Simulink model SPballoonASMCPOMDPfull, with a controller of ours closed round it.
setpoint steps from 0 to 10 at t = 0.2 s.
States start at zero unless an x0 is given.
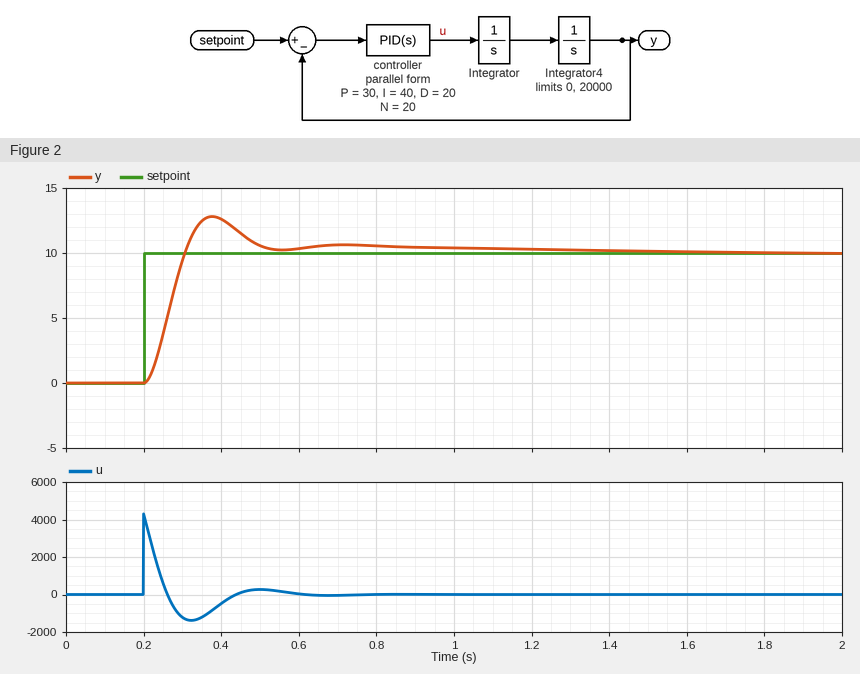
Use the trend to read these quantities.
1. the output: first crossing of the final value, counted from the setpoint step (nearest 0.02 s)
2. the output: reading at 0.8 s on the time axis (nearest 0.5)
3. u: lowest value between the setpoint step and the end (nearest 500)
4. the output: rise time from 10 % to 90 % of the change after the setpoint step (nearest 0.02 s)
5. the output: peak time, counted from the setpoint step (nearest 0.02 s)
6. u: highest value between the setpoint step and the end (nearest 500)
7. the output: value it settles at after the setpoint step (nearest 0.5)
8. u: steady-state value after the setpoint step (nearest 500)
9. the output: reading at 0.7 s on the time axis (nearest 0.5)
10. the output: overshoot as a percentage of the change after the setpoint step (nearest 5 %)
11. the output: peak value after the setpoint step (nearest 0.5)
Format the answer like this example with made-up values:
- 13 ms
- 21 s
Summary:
- 0.10 s
- 10.5
- -1500
- 0.08 s
- 0.18 s
- 4500
- 10.0
- 0
- 10.5
- 30 %
- 13.0
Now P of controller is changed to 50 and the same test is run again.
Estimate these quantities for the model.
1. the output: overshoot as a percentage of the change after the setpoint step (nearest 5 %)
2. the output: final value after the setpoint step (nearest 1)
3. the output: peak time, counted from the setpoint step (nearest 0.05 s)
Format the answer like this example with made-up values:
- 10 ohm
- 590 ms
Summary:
- 35 %
- 10
- 0.15 s
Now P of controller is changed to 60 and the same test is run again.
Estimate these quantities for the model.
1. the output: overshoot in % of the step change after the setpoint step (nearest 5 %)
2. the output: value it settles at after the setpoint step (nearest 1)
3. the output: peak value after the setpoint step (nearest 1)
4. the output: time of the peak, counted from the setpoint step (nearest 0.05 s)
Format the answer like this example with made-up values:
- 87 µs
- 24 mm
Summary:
- 35 %
- 10
- 14
- 0.15 s
